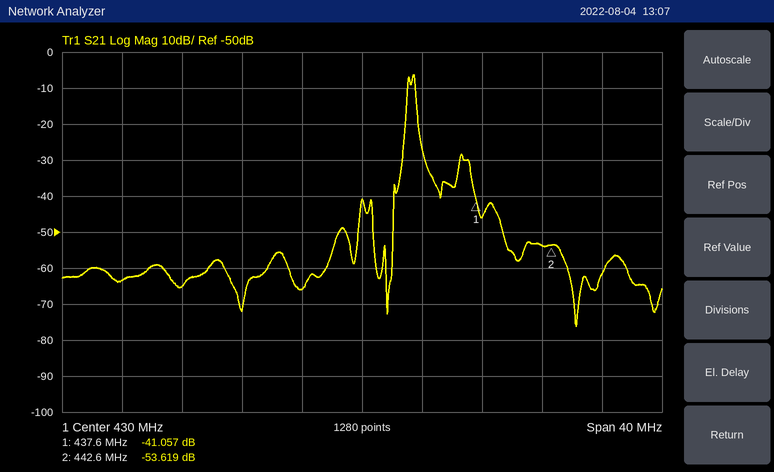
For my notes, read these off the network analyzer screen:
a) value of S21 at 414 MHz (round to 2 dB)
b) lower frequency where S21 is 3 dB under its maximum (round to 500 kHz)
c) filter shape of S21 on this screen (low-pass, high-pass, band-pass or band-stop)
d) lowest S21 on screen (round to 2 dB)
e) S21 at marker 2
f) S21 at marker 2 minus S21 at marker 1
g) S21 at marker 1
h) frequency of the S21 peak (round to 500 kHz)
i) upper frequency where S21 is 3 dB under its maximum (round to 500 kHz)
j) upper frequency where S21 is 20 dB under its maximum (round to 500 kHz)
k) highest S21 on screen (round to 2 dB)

-64 dB
433.0 MHz
band-pass
-76 dB
-53.619 dB
-12.562 dB
-41.057 dB
433.5 MHz
433.5 MHz
434.0 MHz
-6 dB
